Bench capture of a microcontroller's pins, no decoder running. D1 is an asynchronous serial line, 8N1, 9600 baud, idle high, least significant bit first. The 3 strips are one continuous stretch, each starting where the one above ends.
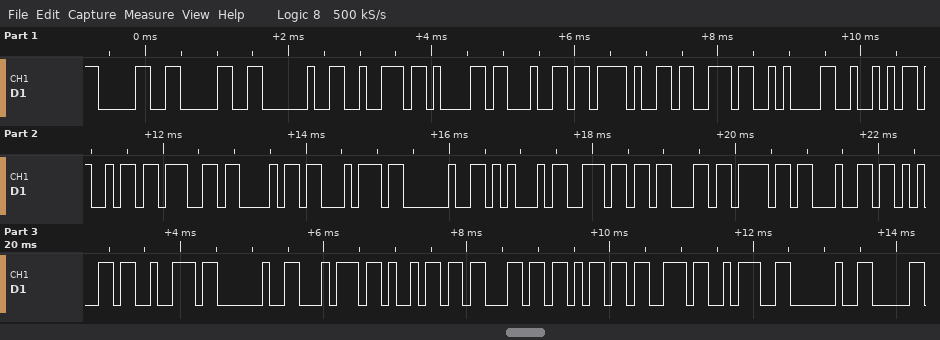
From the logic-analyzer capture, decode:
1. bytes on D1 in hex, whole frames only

30 30 20 72 61 64 2F 73 0A 52 69 67 68 74 20 45 6E 63 6F 64 65 72 20 74 69 63 6B 73 3A 20
